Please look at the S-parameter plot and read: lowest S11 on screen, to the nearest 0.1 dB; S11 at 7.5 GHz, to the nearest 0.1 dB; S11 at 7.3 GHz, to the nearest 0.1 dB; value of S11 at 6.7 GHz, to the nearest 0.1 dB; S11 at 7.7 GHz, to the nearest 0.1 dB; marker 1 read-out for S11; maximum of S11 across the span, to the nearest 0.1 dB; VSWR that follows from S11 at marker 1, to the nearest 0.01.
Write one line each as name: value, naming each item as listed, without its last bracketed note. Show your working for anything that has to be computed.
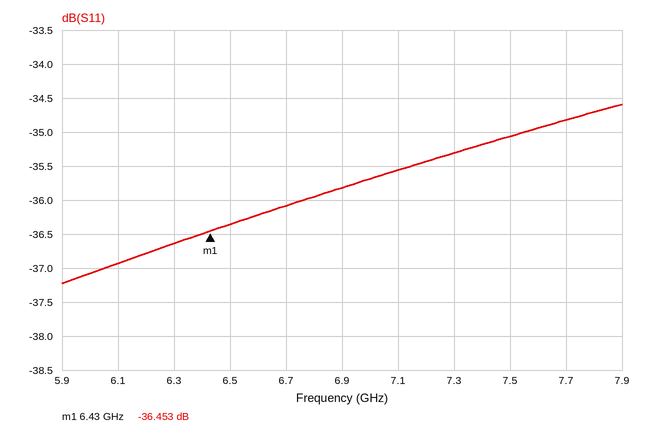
lowest S11 on screen, to the nearest 0.1 dB: -37.2 dB
S11 at 7.5 GHz, to the nearest 0.1 dB: -35.1 dB
S11 at 7.3 GHz, to the nearest 0.1 dB: -35.3 dB
value of S11 at 6.7 GHz, to the nearest 0.1 dB: -36.1 dB
S11 at 7.7 GHz, to the nearest 0.1 dB: -34.8 dB
marker 1 read-out for S11: -36.453 dB
maximum of S11 across the span, to the nearest 0.1 dB: -34.6 dB
VSWR that follows from S11 at marker 1, to the nearest 0.01: (1 + 0.0150)/(1 − 0.0150) ≈ 1.03
